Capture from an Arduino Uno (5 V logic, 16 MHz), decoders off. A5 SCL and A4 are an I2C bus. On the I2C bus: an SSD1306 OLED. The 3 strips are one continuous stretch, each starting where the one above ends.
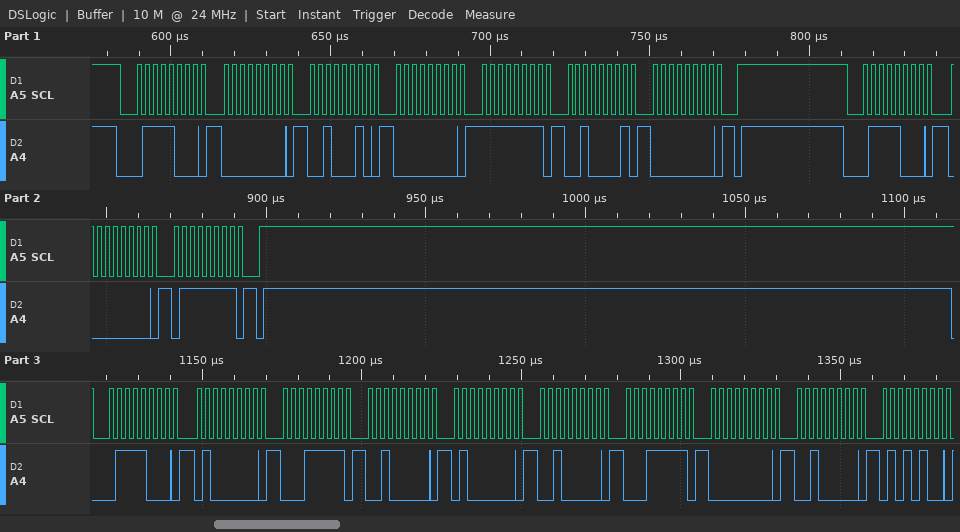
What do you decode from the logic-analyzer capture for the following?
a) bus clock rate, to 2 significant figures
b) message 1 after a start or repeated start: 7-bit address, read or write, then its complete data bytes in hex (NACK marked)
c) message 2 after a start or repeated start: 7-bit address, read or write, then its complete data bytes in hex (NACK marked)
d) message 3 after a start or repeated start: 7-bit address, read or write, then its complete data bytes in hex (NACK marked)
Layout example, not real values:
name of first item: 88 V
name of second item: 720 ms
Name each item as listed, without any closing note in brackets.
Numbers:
bus clock rate, to 2 significant figures: 400 kHz
message 1 after a start or repeated start: 7-bit address, read or write, then its complete data bytes in hex: 0x3C write: 00 22 00 FF 21 00
message 2 after a start or repeated start: 7-bit address, read or write, then its complete data bytes in hex: 0x3C write: 00 7F
message 3 after a start or repeated start: 7-bit address, read or write, then its complete data bytes in hex: 0x3C write: 40 1F 20 40 20 1F 00 20 54
